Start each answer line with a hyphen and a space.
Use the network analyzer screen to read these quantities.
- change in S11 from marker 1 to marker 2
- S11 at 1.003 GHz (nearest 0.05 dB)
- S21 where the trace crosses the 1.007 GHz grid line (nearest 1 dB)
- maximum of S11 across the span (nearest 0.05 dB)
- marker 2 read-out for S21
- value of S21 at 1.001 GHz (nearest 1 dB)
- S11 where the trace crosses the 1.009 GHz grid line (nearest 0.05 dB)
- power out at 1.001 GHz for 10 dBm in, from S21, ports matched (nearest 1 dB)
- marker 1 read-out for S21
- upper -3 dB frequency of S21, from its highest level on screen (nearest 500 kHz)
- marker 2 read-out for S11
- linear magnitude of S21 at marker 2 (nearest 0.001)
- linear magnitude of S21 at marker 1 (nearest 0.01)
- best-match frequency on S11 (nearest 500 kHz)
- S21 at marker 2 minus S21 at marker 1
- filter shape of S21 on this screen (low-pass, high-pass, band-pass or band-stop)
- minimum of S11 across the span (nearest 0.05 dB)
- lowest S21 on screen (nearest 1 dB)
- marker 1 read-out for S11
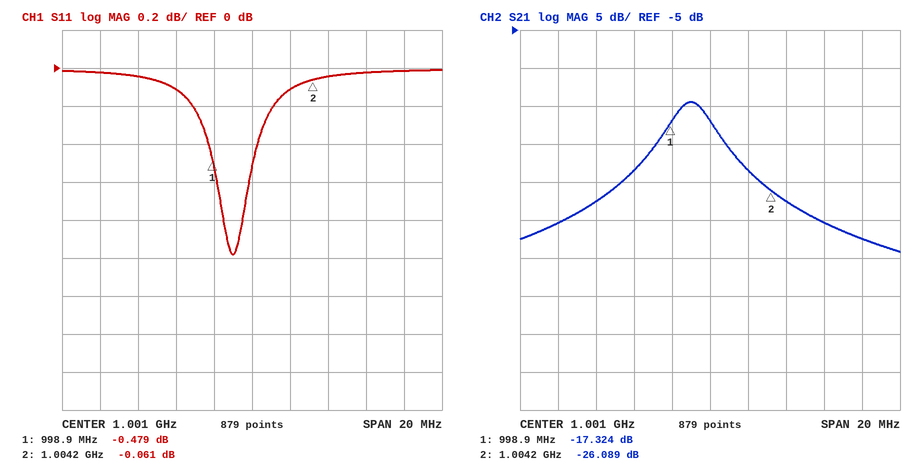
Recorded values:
- 0.418 dB
- -0.10 dB
- -30 dB
- 0.00 dB
- -26.089 dB
- -17 dB
- 0.00 dB
- -7 dBm
- -17.324 dB
- 1.0010 GHz
- -0.061 dB
- 0.050
- 0.14
- 1.0000 GHz
- -8.765 dB
- band-pass
- -1.00 dB
- -34 dB
- -0.479 dB
